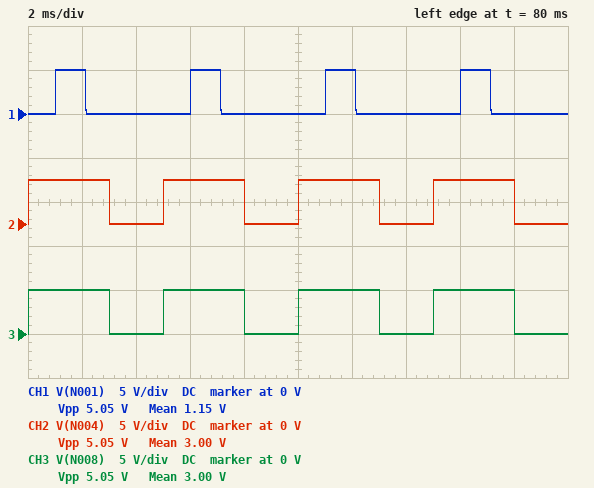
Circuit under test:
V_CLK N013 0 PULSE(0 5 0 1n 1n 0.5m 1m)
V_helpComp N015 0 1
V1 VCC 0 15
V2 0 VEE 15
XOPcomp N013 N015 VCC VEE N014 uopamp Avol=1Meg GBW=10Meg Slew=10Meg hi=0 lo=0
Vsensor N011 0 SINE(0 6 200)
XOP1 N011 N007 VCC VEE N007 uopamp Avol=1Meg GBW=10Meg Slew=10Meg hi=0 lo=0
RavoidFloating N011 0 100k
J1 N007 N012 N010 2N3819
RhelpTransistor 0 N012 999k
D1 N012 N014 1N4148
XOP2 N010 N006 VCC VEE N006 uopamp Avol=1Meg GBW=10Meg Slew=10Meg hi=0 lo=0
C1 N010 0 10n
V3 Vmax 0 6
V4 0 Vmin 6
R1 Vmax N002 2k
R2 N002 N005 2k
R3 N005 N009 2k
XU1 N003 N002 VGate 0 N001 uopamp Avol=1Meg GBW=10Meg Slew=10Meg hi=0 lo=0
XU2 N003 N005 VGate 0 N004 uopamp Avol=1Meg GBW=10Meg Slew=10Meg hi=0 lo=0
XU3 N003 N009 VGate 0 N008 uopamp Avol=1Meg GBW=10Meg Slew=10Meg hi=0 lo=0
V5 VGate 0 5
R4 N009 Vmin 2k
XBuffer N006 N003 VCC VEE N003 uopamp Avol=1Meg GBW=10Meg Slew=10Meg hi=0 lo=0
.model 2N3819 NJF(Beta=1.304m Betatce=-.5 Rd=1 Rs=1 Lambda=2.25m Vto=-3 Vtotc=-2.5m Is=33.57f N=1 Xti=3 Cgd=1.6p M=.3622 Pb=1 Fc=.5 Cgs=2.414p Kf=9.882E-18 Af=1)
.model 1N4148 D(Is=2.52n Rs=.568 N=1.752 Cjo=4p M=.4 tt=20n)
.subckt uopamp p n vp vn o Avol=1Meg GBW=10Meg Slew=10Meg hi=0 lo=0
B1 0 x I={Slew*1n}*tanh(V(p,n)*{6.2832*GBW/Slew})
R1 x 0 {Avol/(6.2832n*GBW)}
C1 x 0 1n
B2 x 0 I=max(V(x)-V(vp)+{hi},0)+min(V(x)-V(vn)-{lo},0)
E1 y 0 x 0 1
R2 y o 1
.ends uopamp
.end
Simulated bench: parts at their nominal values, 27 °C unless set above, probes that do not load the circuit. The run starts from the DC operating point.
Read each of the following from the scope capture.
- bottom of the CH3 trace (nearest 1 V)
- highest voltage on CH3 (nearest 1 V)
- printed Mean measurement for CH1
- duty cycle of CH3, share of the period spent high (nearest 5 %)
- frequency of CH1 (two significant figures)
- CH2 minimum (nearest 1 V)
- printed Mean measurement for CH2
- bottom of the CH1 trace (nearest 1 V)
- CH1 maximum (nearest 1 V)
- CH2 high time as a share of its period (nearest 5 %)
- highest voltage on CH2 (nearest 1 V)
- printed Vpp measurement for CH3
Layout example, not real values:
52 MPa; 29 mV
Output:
0 V; 5 V; 1.15 V; 60 %; 200 Hz; 0 V; 3.00 V; 0 V; 5 V; 60 %; 5 V; 5.05 V
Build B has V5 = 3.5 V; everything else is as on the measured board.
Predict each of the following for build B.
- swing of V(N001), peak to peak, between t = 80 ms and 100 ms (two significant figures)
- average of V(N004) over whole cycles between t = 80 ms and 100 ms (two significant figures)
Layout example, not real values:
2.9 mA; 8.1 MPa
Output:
3.5 V; 2.1 V
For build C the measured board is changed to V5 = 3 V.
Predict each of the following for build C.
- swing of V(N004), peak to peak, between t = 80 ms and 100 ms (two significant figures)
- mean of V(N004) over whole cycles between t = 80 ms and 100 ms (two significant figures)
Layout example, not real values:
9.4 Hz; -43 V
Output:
3.0 V; 1.8 V
